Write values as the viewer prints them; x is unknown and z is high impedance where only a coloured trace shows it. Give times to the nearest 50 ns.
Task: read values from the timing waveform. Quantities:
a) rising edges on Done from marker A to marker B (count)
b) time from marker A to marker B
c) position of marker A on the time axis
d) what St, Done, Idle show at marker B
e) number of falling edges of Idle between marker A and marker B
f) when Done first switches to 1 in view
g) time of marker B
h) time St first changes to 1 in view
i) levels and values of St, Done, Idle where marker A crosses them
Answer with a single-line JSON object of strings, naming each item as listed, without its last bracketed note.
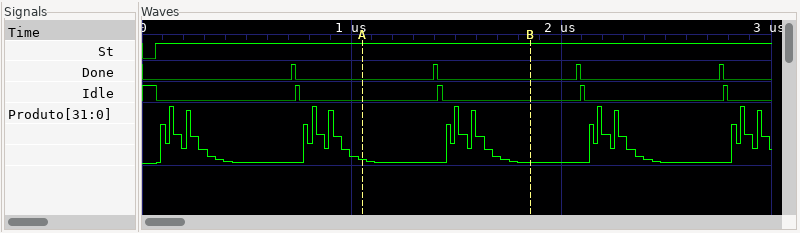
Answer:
{"rising edges on Done from marker A to marker B": "1", "time from marker A to marker B": "800 ns", "position of marker A on the time axis": "1050 ns", "what St, Done, Idle show at marker B": "St=1, Done=0, Idle=0", "number of falling edges of Idle between marker A and marker B": "1", "when Done first switches to 1 in view": "700 ns", "time of marker B": "1850 ns", "time St first changes to 1 in view": "50 ns", "levels and values of St, Done, Idle where marker A crosses them": "St=1, Done=0, Idle=0"}
